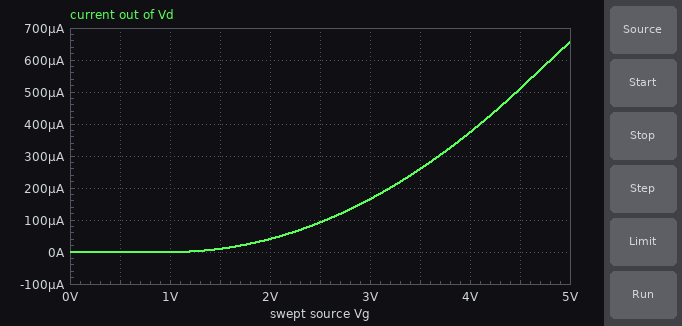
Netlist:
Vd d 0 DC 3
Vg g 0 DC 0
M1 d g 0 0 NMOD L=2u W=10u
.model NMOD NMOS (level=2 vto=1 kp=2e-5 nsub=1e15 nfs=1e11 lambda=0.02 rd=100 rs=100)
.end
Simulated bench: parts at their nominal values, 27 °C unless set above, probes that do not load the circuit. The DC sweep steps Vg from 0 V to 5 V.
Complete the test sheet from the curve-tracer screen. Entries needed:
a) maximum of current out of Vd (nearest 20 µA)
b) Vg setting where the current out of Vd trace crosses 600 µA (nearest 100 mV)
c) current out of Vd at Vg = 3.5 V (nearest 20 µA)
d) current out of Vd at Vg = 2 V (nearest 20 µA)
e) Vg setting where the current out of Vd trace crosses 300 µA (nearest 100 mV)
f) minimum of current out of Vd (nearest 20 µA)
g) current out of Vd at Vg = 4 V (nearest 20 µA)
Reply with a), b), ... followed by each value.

a) 660 µA
b) 4.8 V
c) 260 µA
d) 40 µA
e) 3.7 V
f) 0 A
g) 380 µA
